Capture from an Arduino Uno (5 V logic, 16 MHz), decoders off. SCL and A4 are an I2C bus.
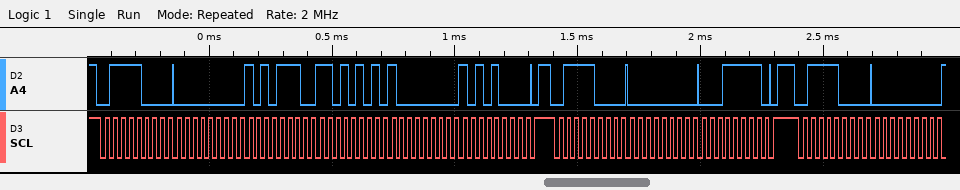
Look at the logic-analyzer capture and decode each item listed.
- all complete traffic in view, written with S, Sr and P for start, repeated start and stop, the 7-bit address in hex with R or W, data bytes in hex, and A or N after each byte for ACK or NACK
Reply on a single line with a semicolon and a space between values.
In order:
S 3CW A 00 A AE A D5 A 80 A A8 A P S 3CW A 00 A 1F A P S 3CW A 00 A
